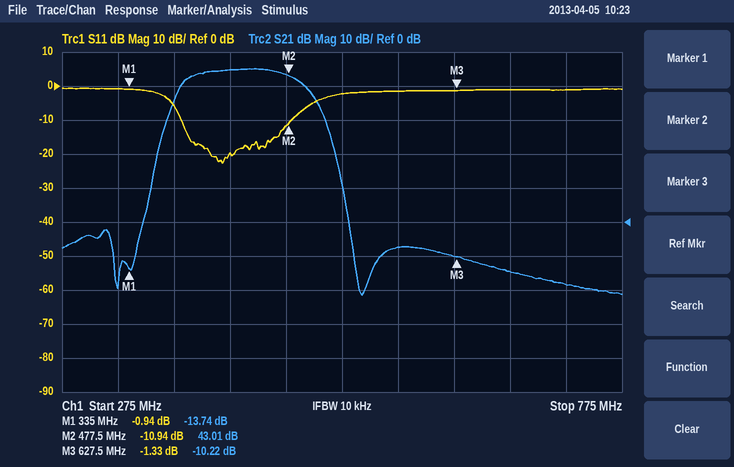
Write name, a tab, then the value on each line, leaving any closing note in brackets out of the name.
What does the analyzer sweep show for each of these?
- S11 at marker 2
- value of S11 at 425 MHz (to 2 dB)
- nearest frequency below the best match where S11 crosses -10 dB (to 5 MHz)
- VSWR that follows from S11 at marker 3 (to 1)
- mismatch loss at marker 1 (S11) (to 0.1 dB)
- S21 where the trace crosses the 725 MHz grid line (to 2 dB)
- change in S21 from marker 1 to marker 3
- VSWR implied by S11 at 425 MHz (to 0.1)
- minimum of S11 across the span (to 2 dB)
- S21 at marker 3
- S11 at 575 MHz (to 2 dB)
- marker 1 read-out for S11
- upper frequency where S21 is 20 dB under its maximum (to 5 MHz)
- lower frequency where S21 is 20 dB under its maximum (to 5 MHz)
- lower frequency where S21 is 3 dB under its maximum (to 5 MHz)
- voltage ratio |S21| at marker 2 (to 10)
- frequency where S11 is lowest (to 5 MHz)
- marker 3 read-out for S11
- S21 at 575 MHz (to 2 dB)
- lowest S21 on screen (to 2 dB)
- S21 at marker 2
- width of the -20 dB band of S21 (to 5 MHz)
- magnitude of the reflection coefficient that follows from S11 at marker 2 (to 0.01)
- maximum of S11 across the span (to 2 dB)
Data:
S11 at marker 2	-10.94 dB
value of S11 at 425 MHz	-20 dB
nearest frequency below the best match where S11 crosses -10 dB	380 MHz
VSWR that follows from S11 at marker 3	13
mismatch loss at marker 1 (S11)	7.1 dB
S21 where the trace crosses the 725 MHz grid line	-18 dB
change in S21 from marker 1 to marker 3	3.52 dB
VSWR implied by S11 at 425 MHz	1.2
minimum of S11 across the span	-22 dB
S21 at marker 3	-10.22 dB
S11 at 575 MHz	-2 dB
marker 1 read-out for S11	-0.94 dB
upper frequency where S21 is 20 dB under its maximum	515 MHz
lower frequency where S21 is 20 dB under its maximum	365 MHz
lower frequency where S21 is 3 dB under its maximum	385 MHz
voltage ratio |S21| at marker 2	140
frequency where S11 is lowest	420 MHz
marker 3 read-out for S11	-1.33 dB
S21 at 575 MHz	-8 dB
lowest S21 on screen	-22 dB
S21 at marker 2	43.01 dB
width of the -20 dB band of S21	150 MHz
magnitude of the reflection coefficient that follows from S11 at marker 2	0.28
maximum of S11 across the span	0 dB
